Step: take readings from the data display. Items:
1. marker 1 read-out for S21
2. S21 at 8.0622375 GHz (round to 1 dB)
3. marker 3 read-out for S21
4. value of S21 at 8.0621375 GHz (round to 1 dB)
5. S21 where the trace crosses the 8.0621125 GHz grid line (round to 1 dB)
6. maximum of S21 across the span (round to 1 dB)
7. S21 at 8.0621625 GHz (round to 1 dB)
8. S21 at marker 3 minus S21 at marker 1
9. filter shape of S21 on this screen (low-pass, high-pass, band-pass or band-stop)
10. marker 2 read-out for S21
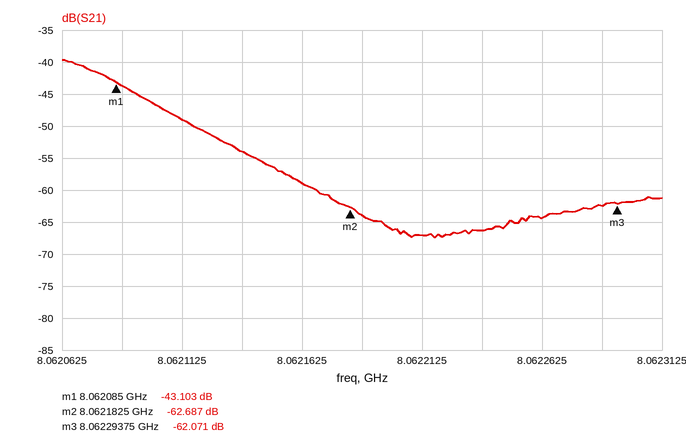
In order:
-43.103 dB
-66 dB
-62.071 dB
-54 dB
-49 dB
-40 dB
-59 dB
-18.968 dB
low-pass
-62.687 dB
